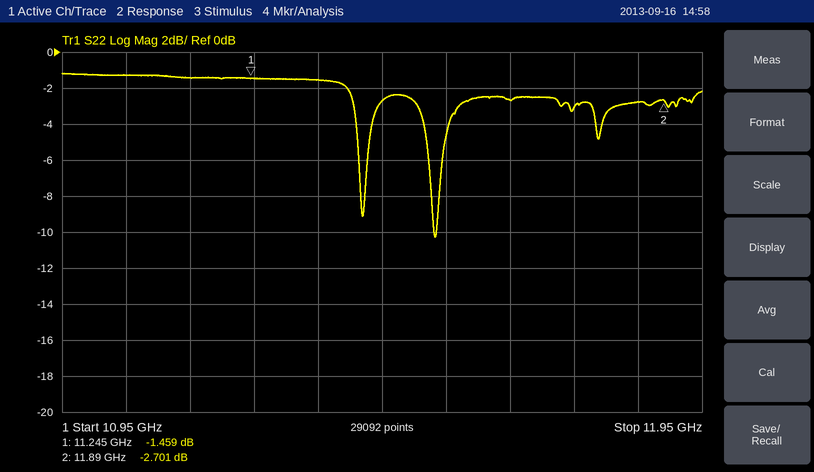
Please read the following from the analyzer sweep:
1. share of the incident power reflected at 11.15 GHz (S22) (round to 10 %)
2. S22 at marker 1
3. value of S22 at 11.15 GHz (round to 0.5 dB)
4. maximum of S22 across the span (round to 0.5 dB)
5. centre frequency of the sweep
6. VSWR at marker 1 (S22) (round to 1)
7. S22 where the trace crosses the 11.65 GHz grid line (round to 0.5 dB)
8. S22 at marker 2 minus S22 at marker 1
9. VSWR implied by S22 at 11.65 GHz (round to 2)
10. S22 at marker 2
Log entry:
70 %
-1.459 dB
-1.5 dB
-1.0 dB
11.45 GHz
12
-2.5 dB
-1.242 dB
6
-2.701 dB
